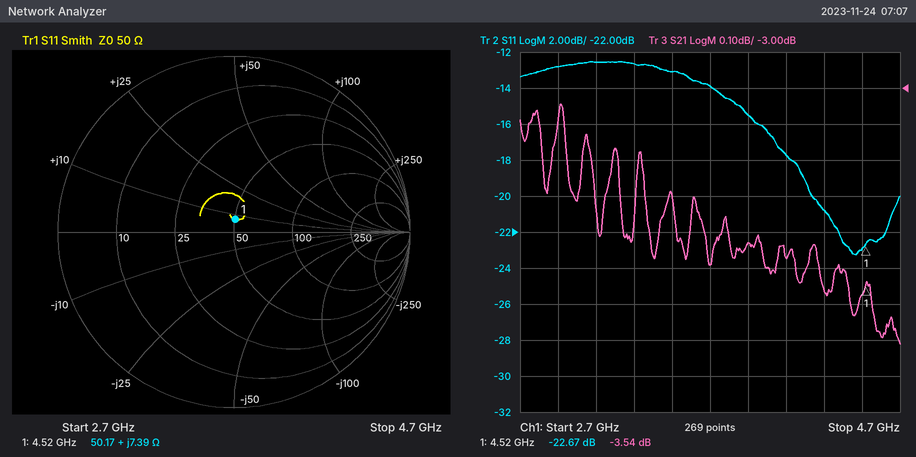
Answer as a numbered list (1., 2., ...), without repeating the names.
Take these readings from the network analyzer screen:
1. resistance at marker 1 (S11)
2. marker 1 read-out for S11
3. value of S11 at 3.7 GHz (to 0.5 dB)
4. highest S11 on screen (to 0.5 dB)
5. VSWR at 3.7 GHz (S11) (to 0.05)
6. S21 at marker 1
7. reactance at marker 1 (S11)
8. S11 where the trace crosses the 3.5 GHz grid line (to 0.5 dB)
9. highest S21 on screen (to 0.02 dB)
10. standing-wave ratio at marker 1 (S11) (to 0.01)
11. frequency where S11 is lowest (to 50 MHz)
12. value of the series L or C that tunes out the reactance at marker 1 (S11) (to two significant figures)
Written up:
1. 50.17 Ω
2. -22.67 dB
3. -14.0 dB
4. -12.5 dB
5. 1.50
6. -3.54 dB
7. +7.39 Ω
8. -13.0 dB
9. -3.04 dB
10. 1.16
11. 4.45 GHz
12. 4.8 pF
